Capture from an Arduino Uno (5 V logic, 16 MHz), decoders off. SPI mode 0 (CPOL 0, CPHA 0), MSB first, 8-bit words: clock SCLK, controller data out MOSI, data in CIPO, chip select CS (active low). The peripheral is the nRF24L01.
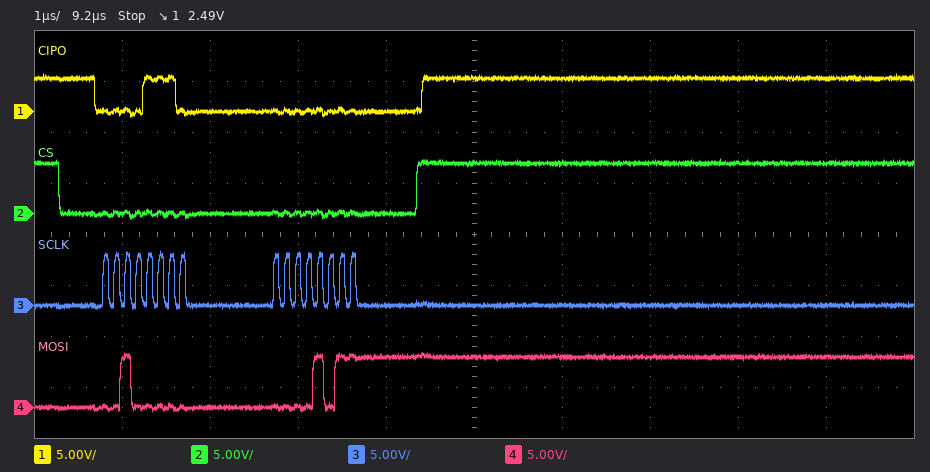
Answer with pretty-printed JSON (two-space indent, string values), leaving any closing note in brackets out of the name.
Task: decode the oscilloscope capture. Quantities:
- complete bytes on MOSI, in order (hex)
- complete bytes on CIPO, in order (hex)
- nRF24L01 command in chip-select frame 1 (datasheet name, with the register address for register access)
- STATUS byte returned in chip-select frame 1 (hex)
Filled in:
{
  "complete bytes on MOSI, in order": "20 0B",
  "complete bytes on CIPO, in order": "0E 00",
  "nRF24L01 command in chip-select frame 1": "W_REGISTER 0x00",
  "STATUS byte returned in chip-select frame 1": "0x0E"
}
